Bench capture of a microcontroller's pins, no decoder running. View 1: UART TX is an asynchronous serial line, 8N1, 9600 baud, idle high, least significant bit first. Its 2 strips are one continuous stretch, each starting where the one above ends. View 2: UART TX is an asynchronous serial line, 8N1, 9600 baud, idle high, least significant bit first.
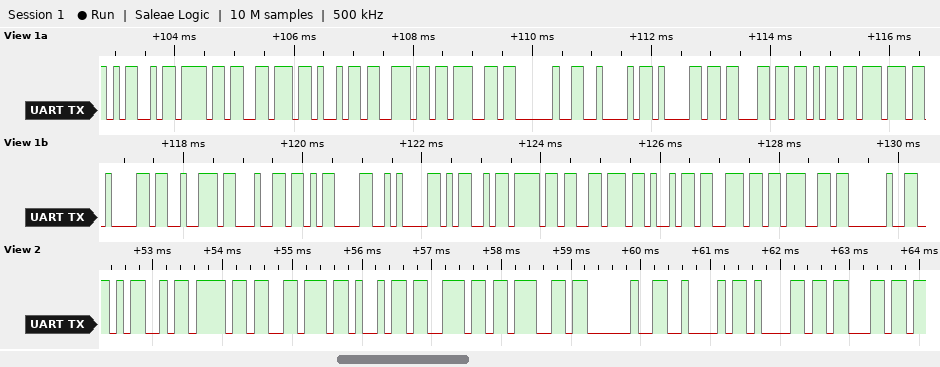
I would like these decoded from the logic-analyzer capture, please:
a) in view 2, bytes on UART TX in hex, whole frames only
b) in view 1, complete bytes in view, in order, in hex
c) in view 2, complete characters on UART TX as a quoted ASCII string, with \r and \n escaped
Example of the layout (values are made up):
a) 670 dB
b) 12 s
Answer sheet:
a) 4D 6F 76 69 6E 67 20 42 61 63
b) 4D 6F 76 69 6E 67 20 42 61 63 6B 77 61 72 64 0D 0A 4D 6F 76 69 6E 67 20
c) "Moving Bac"
